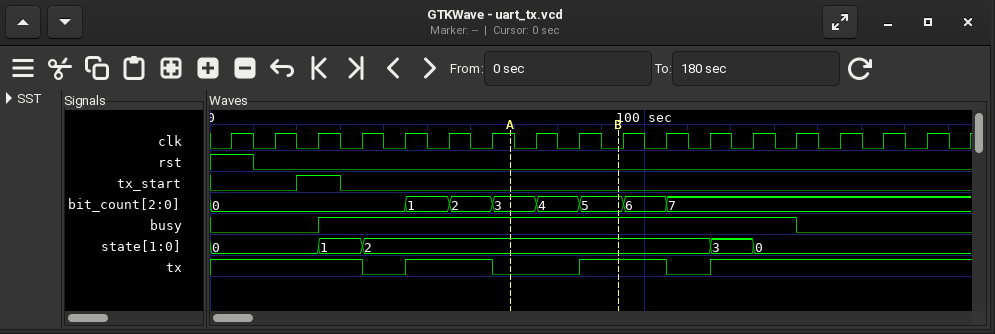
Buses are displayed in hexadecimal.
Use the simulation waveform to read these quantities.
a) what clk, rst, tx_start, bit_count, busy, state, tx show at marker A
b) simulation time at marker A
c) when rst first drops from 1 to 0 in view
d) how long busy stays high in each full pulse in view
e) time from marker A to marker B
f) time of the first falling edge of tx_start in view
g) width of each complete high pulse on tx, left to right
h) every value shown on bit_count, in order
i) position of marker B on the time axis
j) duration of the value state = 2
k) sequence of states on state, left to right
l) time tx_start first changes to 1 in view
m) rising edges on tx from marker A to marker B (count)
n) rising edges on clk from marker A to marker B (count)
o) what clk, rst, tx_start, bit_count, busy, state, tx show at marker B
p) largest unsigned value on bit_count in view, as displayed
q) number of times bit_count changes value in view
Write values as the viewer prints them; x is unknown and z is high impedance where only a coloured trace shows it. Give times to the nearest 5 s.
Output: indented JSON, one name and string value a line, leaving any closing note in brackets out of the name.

{
  "what clk, rst, tx_start, bit_count, busy, state, tx show at marker A": "clk=1, rst=0, tx_start=0, bit_count=3, busy=1, state=2, tx=0",
  "simulation time at marker A": "70 s",
  "when rst first drops from 1 to 0 in view": "10 s",
  "how long busy stays high in each full pulse in view": "110 s",
  "time from marker A to marker B": "25 s",
  "time of the first falling edge of tx_start in view": "30 s",
  "width of each complete high pulse on tx, left to right": "20 s, 20 s",
  "every value shown on bit_count, in order": "0, 1, 2, 3, 4, 5, 6, 7",
  "position of marker B on the time axis": "95 s",
  "duration of the value state = 2": "80 s",
  "sequence of states on state, left to right": "0, 1, 2, 3, 0",
  "time tx_start first changes to 1 in view": "20 s",
  "rising edges on tx from marker A to marker B": "1",
  "rising edges on clk from marker A to marker B": "2",
  "what clk, rst, tx_start, bit_count, busy, state, tx show at marker B": "clk=0, rst=0, tx_start=0, bit_count=5, busy=1, state=2, tx=1",
  "largest unsigned value on bit_count in view, as displayed": "7",
  "number of times bit_count changes value in view": "7"
}
